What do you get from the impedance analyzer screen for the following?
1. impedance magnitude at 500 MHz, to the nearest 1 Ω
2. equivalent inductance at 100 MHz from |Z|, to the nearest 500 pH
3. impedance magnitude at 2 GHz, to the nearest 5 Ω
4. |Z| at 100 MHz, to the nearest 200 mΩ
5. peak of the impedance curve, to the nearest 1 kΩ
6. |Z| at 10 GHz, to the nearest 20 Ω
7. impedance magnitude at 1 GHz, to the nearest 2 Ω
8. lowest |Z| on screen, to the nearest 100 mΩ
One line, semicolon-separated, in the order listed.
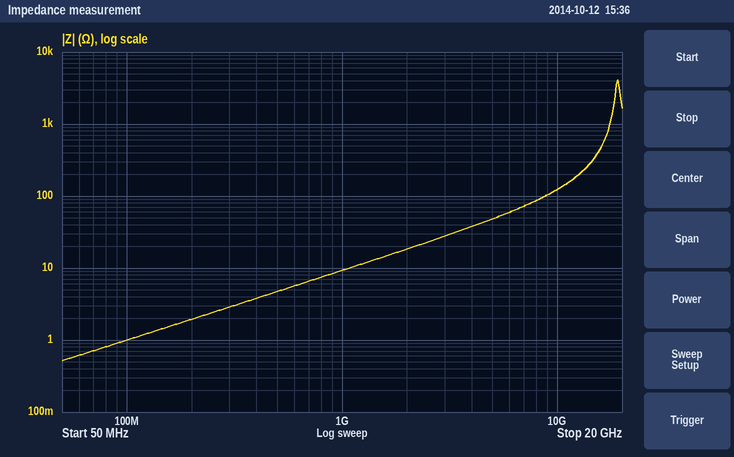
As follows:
5 Ω; 1.5 nH; 20 Ω; 1.0 Ω; 4 kΩ; 120 Ω; 10 Ω; 500 mΩ
